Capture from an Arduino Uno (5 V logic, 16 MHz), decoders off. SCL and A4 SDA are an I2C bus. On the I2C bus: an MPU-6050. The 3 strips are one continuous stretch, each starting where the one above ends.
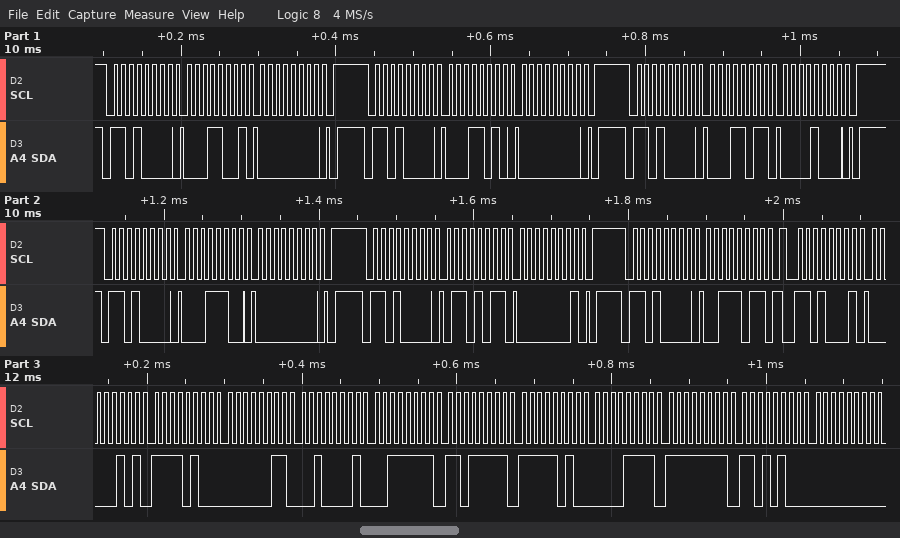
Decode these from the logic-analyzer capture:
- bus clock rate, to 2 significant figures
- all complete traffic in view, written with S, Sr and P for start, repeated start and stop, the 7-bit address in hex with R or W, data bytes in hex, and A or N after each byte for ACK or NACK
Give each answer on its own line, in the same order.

100 kHz
S 68W A 19 A 00 A P S 68W A 1A A 00 A P S 68W A 1B A 08 A P S 68W A 1C A 00 A P S 68W A 6B A 01 A P S 68W A 3B A Sr 68R A 05 A F4 A 03 A 21 A 3F A DF A FA A 0F A FF A D4 A 00 A
